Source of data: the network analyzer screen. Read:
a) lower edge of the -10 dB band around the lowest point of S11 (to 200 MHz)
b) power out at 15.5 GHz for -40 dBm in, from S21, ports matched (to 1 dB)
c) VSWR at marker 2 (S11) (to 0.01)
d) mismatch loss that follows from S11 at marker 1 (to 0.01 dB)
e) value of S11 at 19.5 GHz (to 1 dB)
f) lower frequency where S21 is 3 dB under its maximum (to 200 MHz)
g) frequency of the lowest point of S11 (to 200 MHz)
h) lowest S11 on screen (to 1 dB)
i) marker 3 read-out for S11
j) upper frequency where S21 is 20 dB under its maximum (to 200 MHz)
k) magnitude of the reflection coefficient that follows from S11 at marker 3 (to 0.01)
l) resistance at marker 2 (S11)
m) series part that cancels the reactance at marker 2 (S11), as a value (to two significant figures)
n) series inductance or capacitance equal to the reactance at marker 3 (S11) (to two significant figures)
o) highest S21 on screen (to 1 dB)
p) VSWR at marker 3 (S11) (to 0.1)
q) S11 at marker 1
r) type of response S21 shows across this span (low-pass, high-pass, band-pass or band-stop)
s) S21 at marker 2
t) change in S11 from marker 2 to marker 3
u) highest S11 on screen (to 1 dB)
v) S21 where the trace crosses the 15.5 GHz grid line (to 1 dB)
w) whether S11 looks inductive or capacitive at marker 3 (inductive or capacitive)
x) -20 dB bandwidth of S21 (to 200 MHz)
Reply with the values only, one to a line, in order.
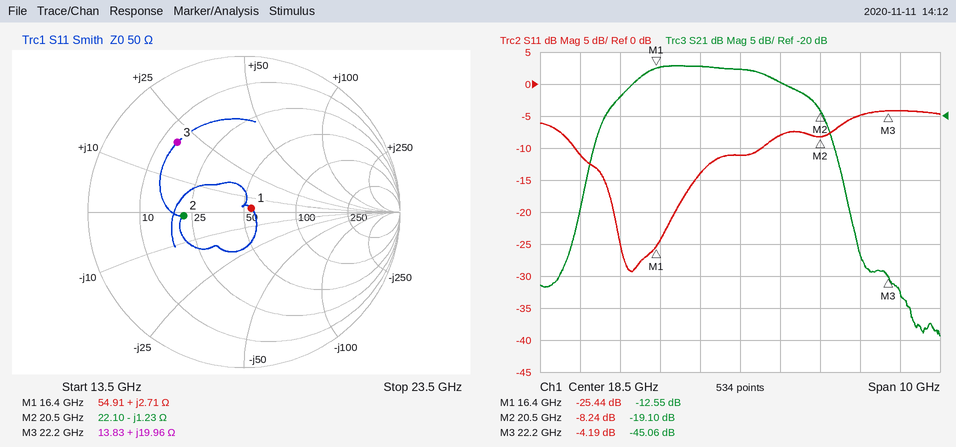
14.4 GHz
-57 dBm
2.26
0.01 dB
-8 dB
15.8 GHz
15.8 GHz
-29 dB
-4.19 dB
21.2 GHz
0.62
22.10 Ω
9.5 pH
140 pH
-12 dB
4.2
-25.44 dB
band-pass
-19.10 dB
4.05 dB
-4 dB
-17 dB
inductive
6.6 GHz
